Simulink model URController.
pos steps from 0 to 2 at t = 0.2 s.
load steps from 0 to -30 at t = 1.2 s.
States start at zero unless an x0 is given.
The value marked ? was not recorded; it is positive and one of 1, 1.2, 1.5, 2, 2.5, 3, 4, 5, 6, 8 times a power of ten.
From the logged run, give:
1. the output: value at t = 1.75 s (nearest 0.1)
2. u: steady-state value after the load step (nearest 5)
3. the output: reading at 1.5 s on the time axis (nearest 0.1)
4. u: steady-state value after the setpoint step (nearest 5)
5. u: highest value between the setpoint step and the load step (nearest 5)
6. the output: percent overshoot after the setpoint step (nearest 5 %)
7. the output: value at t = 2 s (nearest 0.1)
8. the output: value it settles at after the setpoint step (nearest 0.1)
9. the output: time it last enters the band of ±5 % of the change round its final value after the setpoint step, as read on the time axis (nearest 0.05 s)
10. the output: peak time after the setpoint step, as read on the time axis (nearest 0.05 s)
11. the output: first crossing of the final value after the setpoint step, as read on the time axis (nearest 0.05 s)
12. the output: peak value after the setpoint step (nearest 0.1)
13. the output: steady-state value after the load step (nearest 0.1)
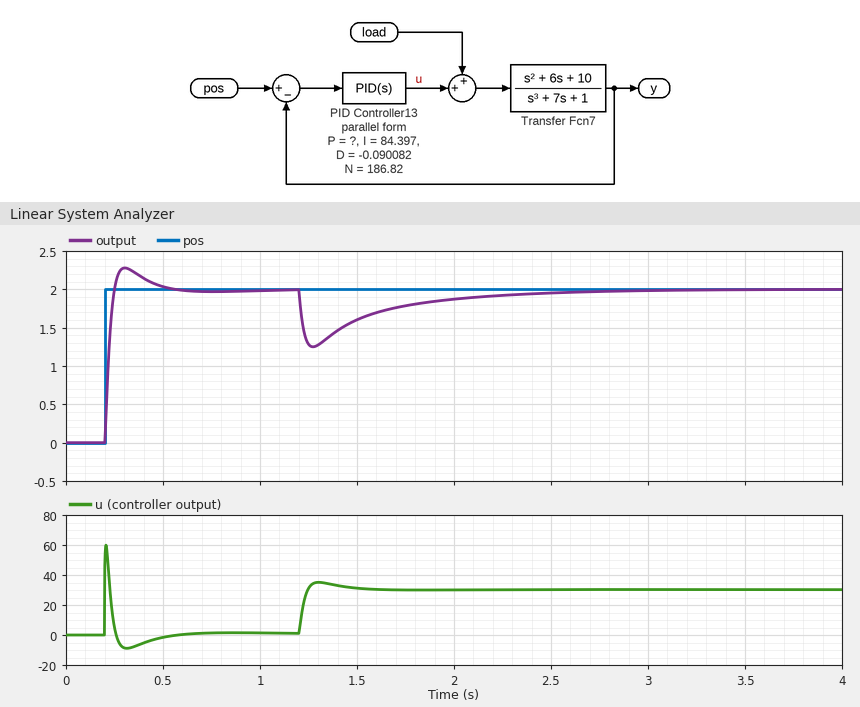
1.8
30
1.6
0
60
15 %
1.9
2.0
0.45 s
0.30 s
0.25 s
2.3
2.0
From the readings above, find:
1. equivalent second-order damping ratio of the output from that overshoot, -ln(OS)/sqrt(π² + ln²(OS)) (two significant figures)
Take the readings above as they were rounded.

0.52
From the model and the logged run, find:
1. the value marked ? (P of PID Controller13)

40
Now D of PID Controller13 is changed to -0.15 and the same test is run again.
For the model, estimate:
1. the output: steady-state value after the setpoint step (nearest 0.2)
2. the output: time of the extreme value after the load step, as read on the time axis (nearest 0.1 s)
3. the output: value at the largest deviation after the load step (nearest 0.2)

2.0
1.3 s
1.2
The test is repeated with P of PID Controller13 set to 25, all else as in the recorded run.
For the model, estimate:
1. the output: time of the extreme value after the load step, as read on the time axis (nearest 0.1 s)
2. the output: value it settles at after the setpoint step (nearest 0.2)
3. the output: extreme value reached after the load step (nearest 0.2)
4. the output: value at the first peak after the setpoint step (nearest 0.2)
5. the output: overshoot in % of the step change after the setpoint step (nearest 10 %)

1.3 s
2.0
0.8
2.4
20 %
